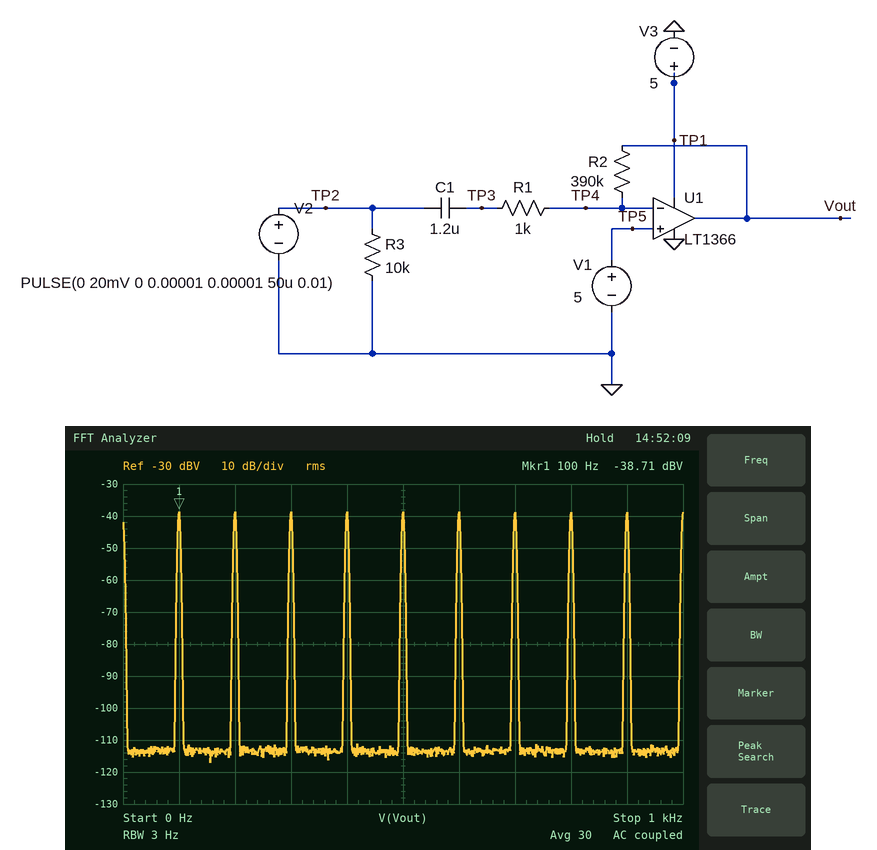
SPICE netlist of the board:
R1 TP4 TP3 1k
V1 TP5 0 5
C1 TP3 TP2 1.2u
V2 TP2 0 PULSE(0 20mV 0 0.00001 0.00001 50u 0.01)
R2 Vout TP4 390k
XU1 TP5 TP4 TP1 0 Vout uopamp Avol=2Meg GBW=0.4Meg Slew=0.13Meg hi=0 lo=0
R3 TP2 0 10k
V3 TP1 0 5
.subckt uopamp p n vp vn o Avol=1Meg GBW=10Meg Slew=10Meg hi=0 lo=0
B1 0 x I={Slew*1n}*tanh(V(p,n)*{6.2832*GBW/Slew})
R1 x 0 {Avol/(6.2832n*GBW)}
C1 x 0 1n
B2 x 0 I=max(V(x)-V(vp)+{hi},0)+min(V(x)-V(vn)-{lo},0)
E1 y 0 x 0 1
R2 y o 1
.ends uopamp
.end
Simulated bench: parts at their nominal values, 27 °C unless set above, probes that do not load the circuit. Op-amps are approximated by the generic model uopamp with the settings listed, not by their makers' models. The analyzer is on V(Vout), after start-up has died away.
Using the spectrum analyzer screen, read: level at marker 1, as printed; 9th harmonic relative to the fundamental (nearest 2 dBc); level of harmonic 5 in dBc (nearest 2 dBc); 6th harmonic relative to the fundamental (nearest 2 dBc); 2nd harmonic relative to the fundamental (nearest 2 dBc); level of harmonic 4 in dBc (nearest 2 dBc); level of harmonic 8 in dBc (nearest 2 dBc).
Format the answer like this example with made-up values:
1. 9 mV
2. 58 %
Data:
1. -38.71 dBV
2. 0 dBc
3. 0 dBc
4. 0 dBc
5. 0 dBc
6. 0 dBc
7. 0 dBc
